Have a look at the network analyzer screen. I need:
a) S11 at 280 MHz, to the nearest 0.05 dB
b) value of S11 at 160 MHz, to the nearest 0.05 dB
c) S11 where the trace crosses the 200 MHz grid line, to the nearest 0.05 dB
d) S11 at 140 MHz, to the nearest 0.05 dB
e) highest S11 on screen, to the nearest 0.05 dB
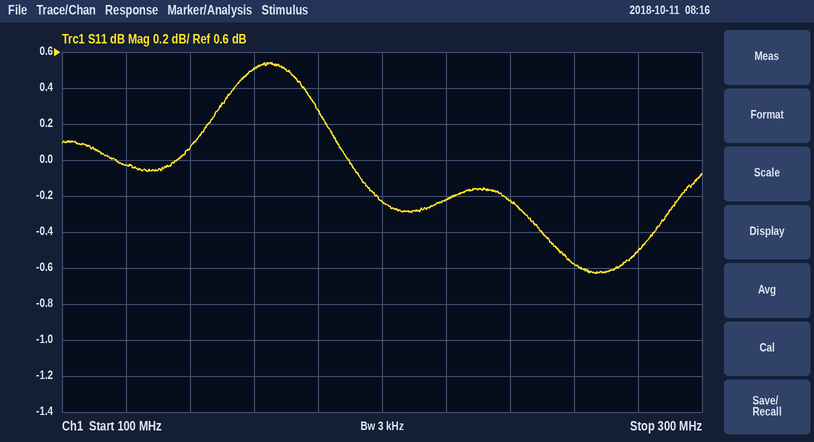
-0.50 dB
0.50 dB
-0.25 dB
0.05 dB
0.55 dB
